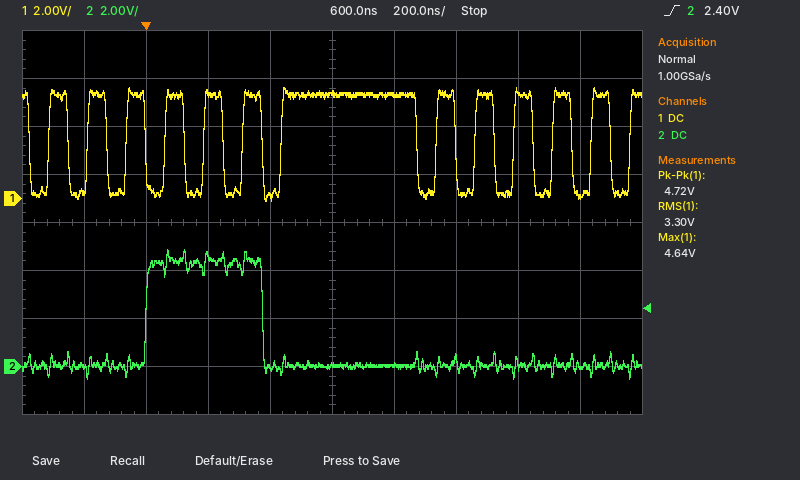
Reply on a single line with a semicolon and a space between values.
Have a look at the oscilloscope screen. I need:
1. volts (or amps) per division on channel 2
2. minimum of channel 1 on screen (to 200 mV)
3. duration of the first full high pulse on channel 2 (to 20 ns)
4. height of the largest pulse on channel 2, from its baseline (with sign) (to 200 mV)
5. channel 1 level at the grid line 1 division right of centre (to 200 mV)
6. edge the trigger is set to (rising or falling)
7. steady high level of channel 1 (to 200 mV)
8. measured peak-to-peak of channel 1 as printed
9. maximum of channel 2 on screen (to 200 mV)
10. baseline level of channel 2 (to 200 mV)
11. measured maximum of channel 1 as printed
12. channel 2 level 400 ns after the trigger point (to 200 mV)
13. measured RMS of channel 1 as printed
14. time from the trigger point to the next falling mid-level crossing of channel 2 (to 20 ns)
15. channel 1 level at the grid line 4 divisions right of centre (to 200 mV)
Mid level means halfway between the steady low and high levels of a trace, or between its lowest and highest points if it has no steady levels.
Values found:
2 V; 0.0 V; 380 ns; +4.8 V; 4.4 V; rising; 4.4 V; 4.72 V; 4.8 V; 0.0 V; 4.64 V; 0.0 V; 3.30 V; 380 ns; 200 mV
